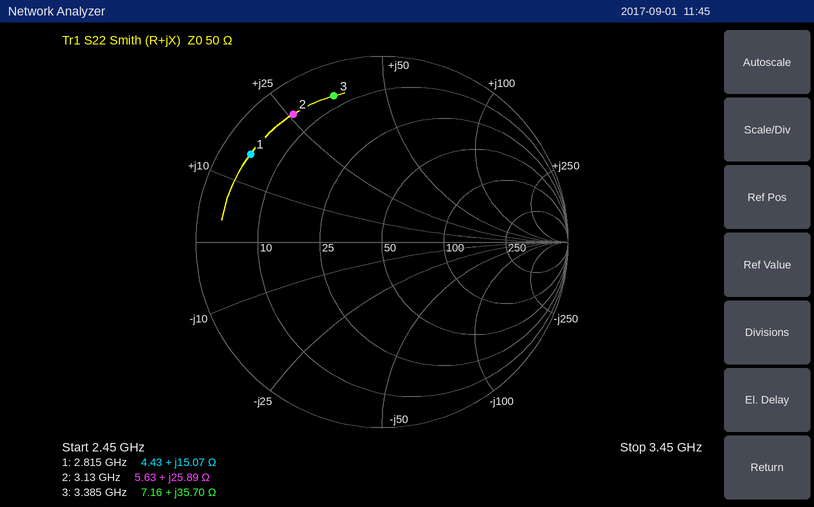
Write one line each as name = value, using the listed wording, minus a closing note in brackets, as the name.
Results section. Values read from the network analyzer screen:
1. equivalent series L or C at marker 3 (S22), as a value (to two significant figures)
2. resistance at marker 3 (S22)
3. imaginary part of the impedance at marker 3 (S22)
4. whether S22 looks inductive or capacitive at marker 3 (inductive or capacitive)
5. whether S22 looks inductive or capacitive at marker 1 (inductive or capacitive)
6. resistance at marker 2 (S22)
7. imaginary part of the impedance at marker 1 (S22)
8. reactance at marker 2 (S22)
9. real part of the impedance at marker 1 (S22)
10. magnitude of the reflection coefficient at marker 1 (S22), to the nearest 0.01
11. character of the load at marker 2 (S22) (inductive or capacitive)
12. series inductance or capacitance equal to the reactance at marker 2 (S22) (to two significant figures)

equivalent series L or C at marker 3 (S22), as a value = 1.7 nH
resistance at marker 3 = 7.16 Ω
imaginary part of the impedance at marker 3 = +35.70 Ω
whether S22 looks inductive or capacitive at marker 3 = inductive
whether S22 looks inductive or capacitive at marker 1 = inductive
resistance at marker 2 = 5.63 Ω
imaginary part of the impedance at marker 1 = +15.07 Ω
reactance at marker 2 = +25.89 Ω
real part of the impedance at marker 1 = 4.43 Ω
magnitude of the reflection coefficient at marker 1 (S22), to the nearest 0.01 = 0.85
character of the load at marker 2 (S22) = inductive
series inductance or capacitance equal to the reactance at marker 2 (S22) = 1.3 nH
